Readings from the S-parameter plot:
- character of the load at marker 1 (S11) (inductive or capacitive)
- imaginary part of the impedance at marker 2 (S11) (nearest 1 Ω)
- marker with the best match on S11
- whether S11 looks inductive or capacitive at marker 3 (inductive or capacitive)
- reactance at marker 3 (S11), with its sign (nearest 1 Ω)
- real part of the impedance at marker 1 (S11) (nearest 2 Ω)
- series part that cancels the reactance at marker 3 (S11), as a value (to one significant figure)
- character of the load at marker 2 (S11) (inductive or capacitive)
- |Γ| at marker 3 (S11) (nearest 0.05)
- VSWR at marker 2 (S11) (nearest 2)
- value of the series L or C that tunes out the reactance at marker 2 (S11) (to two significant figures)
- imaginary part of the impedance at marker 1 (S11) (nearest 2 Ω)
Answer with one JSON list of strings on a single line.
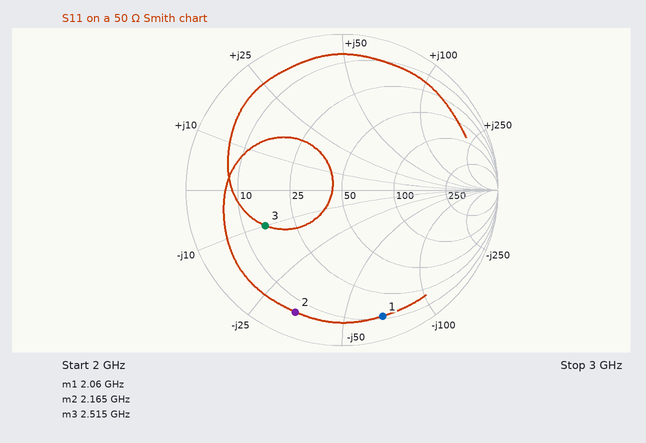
["capacitive", "-34 Ω", "marker 3", "capacitive", "-10 Ω", "12 Ω", "600 pH", "capacitive", "0.55", "12", "2.5 nH", "-68 Ω"]
